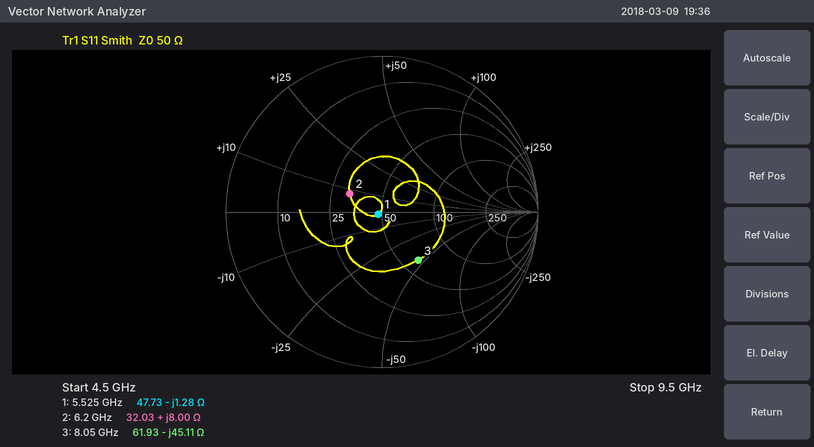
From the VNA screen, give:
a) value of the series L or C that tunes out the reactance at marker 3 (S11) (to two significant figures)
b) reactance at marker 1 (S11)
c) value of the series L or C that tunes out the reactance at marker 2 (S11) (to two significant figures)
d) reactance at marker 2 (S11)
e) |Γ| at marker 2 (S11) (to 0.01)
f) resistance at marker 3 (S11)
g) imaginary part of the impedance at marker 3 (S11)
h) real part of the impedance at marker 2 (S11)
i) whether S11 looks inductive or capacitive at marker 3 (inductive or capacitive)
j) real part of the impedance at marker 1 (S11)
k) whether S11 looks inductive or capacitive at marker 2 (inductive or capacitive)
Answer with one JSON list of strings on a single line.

["890 pH", "-1.28 Ω", "3.2 pF", "+8.00 Ω", "0.24", "61.93 Ω", "-45.11 Ω", "32.03 Ω", "capacitive", "47.73 Ω", "inductive"]
